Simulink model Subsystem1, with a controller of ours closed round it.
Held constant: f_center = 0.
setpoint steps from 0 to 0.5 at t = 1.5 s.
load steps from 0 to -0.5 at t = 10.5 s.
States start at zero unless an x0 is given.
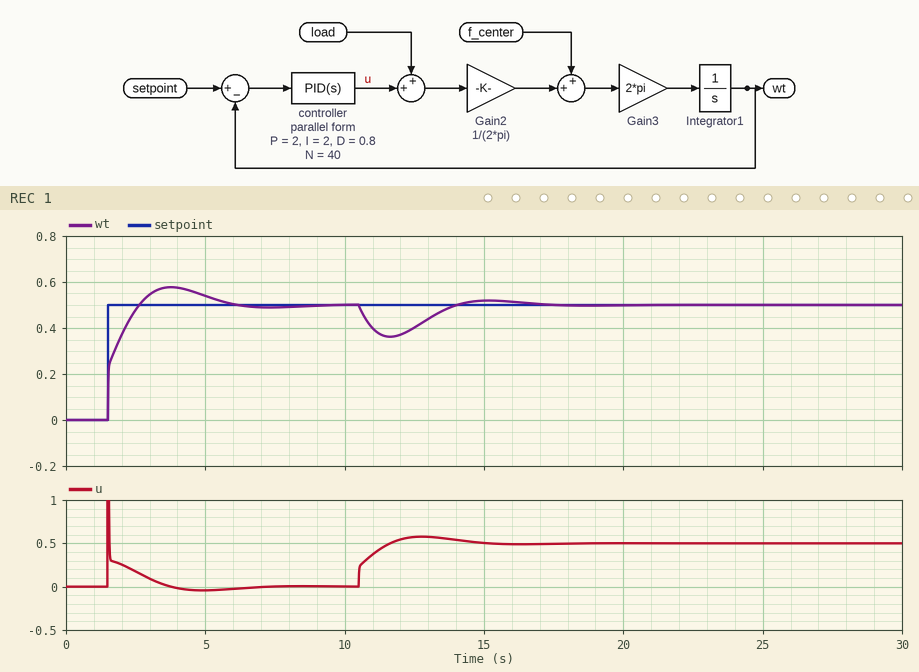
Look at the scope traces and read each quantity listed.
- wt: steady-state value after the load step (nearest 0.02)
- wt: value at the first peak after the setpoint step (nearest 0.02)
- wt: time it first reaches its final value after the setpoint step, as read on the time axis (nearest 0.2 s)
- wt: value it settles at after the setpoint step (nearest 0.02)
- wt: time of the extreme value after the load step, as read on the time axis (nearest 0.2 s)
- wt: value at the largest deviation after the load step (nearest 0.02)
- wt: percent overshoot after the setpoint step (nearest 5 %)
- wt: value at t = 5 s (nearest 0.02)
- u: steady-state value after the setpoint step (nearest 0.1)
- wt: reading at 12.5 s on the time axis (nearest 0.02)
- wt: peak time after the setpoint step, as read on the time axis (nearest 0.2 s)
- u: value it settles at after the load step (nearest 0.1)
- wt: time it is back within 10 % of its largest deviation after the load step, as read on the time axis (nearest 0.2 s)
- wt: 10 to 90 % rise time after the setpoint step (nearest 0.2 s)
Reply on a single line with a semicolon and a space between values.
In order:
0.50; 0.58; 2.6 s; 0.50; 11.6 s; 0.36; 15 %; 0.54; 0.0; 0.40; 3.8 s; 0.5; 16.0 s; 0.8 s
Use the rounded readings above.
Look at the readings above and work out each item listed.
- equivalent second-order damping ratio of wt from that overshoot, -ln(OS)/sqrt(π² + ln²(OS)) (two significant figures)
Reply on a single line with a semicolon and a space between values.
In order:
0.52
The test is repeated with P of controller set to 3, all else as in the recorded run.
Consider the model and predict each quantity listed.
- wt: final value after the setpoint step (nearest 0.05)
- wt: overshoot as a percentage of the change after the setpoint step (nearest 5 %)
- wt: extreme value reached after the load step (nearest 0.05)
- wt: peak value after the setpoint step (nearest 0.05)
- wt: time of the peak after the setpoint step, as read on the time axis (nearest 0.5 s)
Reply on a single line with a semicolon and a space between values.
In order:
0.50; 10 %; 0.40; 0.55; 3.5 s
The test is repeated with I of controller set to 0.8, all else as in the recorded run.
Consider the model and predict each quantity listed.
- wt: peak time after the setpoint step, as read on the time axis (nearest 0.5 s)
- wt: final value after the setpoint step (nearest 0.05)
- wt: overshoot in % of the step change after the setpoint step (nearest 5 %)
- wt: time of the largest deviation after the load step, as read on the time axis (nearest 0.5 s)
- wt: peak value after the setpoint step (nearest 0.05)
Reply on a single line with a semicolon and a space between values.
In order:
4.5 s; 0.50; 10 %; 12.0 s; 0.55
